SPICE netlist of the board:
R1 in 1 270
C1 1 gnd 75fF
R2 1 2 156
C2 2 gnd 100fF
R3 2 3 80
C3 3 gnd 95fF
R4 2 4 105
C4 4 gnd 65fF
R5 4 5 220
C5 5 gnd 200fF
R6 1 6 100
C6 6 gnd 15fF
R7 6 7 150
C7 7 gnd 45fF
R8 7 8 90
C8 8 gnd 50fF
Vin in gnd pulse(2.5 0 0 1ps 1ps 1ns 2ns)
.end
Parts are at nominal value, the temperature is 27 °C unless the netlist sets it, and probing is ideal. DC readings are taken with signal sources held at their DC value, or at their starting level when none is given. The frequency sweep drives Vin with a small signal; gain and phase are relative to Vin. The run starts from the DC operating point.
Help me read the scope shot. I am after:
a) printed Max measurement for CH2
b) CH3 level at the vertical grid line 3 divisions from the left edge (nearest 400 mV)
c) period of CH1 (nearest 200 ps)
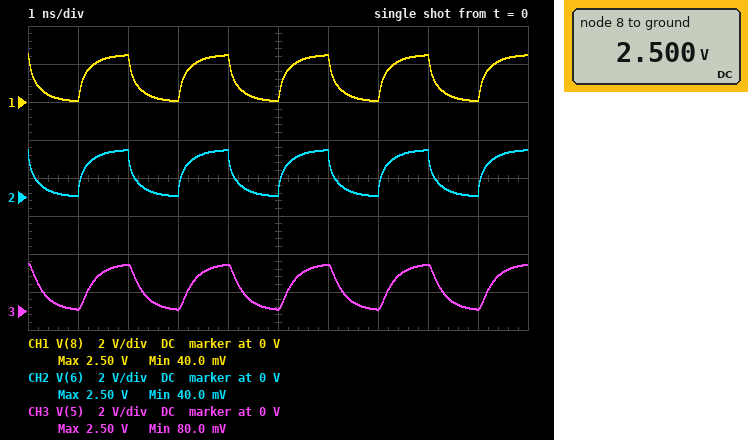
2.50 V
0 V
2.0 ns
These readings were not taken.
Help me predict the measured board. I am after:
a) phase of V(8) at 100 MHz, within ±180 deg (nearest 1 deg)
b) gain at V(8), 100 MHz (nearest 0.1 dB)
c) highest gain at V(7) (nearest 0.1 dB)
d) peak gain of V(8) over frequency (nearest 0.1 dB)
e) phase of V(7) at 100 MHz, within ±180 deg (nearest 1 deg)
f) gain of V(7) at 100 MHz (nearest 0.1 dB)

-7 deg
-0.1 dB
0 dB
0 dB
-7 deg
-0.1 dB
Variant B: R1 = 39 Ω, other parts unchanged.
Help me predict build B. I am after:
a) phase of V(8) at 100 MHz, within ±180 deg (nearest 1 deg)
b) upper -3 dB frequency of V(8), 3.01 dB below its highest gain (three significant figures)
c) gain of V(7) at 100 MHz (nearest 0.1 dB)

-2 deg
3.68 GHz
0 dB
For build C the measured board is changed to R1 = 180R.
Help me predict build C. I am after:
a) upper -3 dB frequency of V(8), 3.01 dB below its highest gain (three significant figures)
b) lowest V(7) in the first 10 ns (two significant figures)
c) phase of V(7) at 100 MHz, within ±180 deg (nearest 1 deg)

1.06 GHz
13 mV
-5 deg
